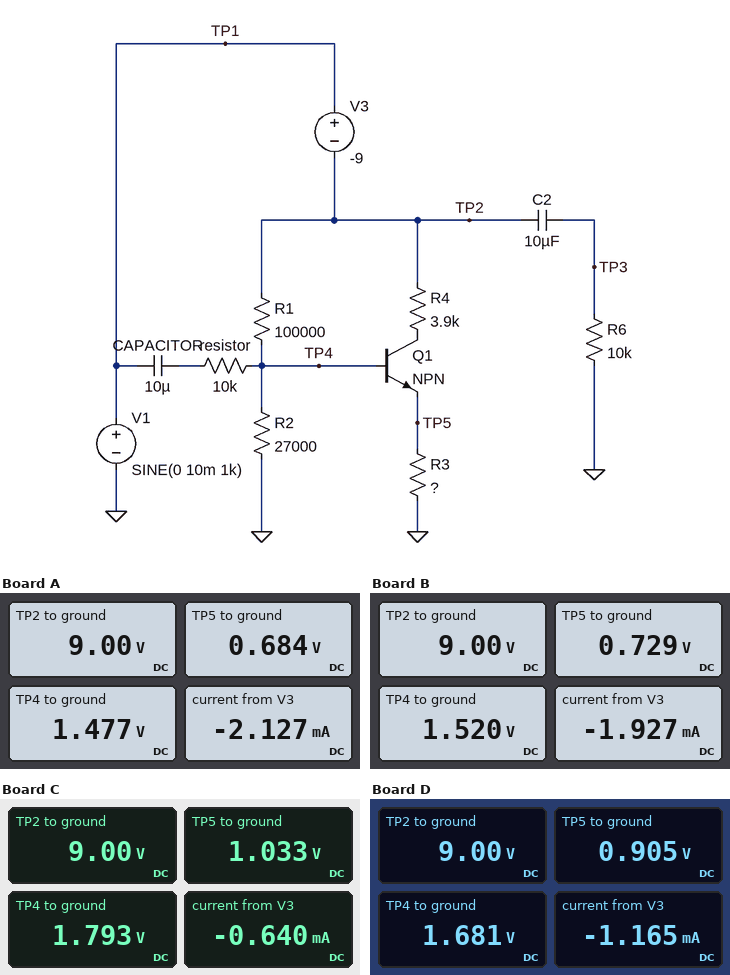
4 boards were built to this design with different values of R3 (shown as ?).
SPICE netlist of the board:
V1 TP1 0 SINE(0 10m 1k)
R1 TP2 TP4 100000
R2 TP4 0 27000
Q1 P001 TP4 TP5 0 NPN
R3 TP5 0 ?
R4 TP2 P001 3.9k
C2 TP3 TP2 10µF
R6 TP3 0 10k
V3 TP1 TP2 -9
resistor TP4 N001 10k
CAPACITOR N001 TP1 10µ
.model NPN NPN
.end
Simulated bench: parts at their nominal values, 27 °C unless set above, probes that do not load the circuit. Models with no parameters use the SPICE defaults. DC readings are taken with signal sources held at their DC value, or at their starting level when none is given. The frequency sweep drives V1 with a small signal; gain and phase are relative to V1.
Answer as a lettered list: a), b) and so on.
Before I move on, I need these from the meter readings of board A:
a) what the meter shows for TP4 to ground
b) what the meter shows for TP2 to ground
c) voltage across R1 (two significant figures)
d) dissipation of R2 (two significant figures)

a) 1.477 V
b) 9.00 V
c) 7.5 V
d) 81 µW
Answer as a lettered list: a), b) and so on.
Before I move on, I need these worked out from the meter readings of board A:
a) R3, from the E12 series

a) 330 Ω
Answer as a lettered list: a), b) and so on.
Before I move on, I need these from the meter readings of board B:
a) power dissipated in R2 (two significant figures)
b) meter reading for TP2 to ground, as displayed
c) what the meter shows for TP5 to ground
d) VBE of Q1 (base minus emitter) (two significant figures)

a) 86 µW
b) 9.00 V
c) 0.729 V
d) 790 mV
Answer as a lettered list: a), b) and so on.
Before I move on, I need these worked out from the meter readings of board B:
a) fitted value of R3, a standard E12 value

a) 390 Ω
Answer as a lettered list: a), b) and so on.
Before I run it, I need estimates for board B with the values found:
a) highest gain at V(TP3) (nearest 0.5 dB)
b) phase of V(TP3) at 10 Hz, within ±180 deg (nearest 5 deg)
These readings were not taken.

a) 0 dB
b) 10 deg
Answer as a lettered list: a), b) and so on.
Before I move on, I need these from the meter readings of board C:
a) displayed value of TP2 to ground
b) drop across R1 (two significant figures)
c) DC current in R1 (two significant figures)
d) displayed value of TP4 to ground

a) 9.00 V
b) 7.2 V
c) 72 µA
d) 1.793 V
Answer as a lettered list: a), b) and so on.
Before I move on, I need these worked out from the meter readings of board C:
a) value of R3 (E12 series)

a) 1.8 kΩ
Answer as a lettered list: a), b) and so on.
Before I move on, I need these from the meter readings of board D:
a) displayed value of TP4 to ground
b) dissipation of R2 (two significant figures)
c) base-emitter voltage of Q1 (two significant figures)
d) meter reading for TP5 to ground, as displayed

a) 1.681 V
b) 100 µW
c) 780 mV
d) 0.905 V
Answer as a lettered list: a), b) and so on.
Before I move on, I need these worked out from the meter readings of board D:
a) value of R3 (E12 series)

a) 820 Ω
